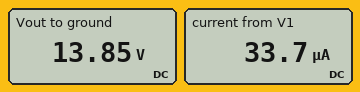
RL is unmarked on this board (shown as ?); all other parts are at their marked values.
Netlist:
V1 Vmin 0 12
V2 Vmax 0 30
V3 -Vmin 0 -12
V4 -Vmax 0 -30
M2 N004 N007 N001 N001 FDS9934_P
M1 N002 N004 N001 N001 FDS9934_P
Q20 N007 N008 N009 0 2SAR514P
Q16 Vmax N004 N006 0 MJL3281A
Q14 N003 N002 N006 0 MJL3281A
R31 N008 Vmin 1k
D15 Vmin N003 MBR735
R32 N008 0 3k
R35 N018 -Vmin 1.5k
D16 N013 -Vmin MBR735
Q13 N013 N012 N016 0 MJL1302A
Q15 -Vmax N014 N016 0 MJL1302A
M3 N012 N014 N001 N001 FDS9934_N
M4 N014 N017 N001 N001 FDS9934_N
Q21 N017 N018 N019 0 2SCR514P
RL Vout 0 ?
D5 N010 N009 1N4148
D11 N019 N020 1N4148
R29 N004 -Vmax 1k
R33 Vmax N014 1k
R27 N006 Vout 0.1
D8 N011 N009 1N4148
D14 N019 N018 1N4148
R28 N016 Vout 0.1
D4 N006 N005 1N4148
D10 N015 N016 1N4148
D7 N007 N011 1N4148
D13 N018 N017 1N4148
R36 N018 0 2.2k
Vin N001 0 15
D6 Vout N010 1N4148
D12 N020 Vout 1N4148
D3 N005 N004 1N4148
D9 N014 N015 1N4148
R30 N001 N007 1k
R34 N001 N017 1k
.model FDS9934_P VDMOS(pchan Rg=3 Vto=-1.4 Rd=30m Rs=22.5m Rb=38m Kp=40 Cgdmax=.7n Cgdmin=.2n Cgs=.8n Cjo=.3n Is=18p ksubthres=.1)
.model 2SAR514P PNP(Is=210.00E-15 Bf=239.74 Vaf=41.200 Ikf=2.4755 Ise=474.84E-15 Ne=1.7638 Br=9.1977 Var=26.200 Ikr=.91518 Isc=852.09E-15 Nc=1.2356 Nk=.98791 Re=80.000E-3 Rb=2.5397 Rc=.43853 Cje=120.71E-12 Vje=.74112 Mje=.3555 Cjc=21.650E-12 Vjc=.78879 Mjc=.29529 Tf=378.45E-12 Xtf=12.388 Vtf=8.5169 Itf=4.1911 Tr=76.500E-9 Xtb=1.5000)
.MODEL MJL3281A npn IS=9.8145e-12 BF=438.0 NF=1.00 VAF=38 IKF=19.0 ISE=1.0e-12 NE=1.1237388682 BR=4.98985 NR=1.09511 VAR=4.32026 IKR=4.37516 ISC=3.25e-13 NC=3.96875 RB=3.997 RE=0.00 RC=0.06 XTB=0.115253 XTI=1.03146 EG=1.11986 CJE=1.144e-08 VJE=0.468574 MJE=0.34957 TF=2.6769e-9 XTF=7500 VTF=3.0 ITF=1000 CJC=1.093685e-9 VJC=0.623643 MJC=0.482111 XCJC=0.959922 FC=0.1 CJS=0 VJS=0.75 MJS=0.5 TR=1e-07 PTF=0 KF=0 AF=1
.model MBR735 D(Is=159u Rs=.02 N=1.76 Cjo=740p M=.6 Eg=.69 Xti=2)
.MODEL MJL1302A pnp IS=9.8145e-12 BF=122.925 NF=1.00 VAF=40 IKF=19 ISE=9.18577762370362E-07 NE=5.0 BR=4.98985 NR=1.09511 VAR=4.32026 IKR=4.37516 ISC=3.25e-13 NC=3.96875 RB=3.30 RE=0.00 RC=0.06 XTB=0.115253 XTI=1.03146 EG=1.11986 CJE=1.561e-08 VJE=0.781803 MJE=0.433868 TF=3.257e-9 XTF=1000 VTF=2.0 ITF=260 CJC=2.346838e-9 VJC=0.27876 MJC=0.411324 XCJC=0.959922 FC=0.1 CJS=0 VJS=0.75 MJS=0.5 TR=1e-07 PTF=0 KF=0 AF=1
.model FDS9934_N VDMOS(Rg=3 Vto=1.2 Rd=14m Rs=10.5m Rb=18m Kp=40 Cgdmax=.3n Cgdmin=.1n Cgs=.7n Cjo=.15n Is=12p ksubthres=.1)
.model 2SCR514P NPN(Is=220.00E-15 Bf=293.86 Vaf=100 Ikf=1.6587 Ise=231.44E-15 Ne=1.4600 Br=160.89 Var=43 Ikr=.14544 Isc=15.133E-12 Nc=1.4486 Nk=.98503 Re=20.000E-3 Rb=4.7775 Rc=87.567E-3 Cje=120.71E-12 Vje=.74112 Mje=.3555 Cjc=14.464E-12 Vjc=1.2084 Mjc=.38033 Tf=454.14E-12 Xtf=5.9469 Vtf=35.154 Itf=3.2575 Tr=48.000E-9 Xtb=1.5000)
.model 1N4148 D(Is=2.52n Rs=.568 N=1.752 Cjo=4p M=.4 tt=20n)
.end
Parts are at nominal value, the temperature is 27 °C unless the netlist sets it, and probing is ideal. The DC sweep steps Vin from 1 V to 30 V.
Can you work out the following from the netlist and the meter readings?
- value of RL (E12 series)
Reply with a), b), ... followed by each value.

a) 3.9 Ω
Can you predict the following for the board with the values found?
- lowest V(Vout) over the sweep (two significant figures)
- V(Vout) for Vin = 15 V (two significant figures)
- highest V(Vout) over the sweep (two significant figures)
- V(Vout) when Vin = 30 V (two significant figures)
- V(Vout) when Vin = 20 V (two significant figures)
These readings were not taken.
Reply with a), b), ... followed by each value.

a) 400 mV
b) 14 V
c) 28 V
d) 28 V
e) 19 V
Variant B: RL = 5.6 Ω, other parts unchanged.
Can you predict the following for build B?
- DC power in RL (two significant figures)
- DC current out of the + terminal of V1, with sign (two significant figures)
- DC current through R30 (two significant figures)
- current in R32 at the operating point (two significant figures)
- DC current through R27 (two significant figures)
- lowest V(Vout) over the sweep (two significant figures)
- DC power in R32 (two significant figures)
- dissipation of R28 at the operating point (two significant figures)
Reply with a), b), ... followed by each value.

a) 35 W
b) -95 µA
c) 2.2 mA
d) 4.0 mA
e) 2.5 A
f) 410 mV
g) 49 mW
h) 21 µW
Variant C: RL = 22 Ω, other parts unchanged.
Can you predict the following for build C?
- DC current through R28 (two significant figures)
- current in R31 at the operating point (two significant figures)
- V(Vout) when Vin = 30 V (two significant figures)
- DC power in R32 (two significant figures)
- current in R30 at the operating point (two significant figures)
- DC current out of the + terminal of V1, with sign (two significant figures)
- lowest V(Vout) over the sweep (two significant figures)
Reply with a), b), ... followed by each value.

a) 14 mA
b) 340 µA
c) 29 V
d) 51 mW
e) 2.0 mA
f) -340 µA
g) 450 mV
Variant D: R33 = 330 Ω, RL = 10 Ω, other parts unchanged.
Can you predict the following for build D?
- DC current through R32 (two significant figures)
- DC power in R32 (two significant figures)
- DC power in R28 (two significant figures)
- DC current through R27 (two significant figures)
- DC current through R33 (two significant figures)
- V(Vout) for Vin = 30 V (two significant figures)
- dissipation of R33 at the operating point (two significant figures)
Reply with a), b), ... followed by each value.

a) 4.1 mA
b) 50 mW
c) 190 µW
d) 1.4 A
e) 43 mA
f) 29 V
g) 620 mW
